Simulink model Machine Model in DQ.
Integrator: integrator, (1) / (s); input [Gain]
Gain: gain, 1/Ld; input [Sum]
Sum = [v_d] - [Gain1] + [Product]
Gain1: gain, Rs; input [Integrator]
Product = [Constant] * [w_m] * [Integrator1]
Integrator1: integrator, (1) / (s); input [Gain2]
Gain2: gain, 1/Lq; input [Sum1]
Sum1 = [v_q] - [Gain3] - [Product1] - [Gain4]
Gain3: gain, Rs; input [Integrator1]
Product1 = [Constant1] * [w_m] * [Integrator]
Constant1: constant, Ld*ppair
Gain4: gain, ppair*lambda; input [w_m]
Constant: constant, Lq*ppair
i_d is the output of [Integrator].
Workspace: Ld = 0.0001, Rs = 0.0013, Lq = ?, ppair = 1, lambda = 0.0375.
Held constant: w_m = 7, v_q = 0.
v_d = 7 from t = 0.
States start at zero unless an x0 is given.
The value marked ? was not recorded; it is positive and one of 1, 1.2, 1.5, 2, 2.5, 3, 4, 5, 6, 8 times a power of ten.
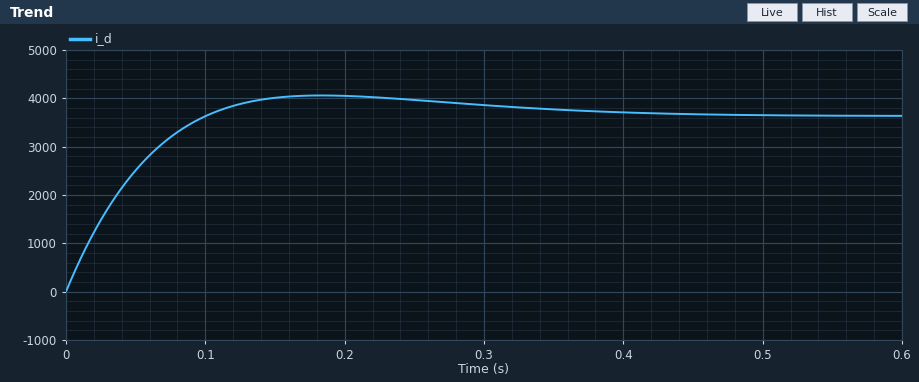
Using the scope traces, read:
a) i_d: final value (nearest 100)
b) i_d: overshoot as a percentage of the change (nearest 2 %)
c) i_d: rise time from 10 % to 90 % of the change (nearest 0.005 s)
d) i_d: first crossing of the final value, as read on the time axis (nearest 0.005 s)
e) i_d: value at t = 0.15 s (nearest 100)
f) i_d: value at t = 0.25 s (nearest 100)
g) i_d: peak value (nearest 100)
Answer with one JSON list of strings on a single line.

["3600", "12 %", "0.075 s", "0.100 s", "4000", "4000", "4100"]
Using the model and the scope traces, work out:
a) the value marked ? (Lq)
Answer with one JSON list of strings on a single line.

["0.00015"]
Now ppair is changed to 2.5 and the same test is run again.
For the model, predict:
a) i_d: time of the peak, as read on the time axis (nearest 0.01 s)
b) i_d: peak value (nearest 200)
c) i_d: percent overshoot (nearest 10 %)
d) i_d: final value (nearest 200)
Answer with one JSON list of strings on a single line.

["0.08 s", "2400", "110 %", "1200"]
